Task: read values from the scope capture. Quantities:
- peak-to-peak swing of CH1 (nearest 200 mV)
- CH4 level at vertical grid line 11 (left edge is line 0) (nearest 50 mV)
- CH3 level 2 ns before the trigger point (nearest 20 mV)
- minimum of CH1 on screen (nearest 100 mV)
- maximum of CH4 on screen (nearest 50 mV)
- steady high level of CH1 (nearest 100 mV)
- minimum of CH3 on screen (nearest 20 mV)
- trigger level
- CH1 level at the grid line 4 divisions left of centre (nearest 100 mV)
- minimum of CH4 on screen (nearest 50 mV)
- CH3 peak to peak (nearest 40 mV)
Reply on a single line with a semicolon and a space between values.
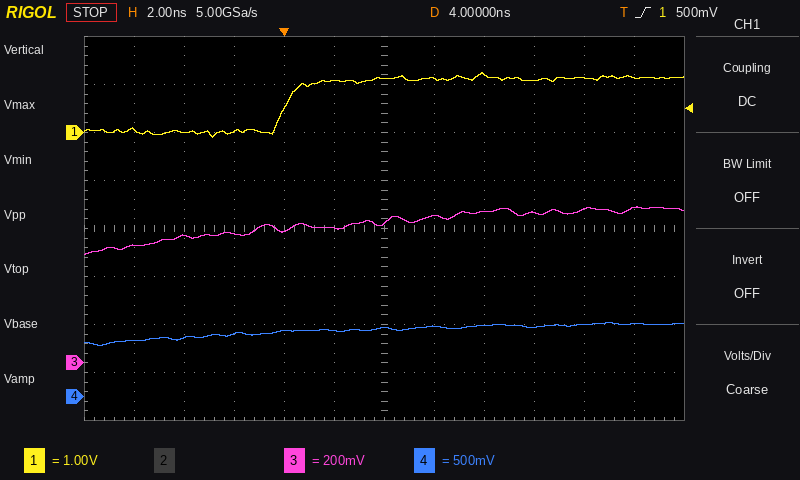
1.4 V; 750 mV; 540 mV; -100 mV; 750 mV; 1.1 V; 460 mV; 500 mV; 0.0 V; 550 mV; 200 mV
